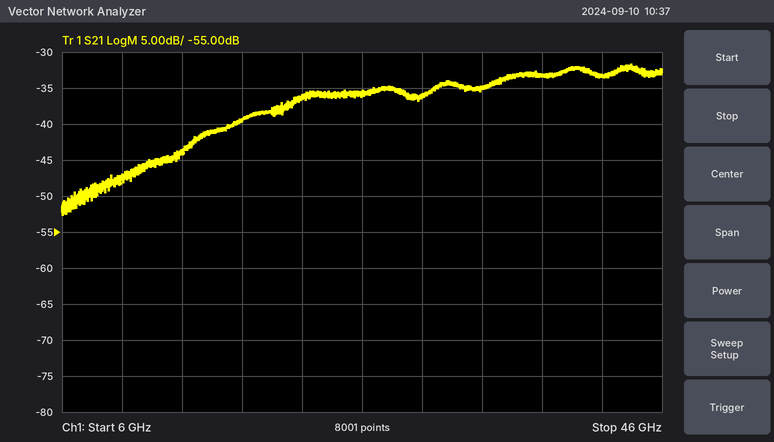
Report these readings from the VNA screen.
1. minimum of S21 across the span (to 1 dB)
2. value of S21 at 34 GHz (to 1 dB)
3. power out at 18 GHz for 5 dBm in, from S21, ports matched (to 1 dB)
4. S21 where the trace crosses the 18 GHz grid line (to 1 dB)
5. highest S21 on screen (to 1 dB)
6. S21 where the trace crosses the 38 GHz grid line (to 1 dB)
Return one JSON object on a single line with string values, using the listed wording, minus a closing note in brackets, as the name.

{"minimum of S21 across the span": "-53 dB", "value of S21 at 34 GHz": "-35 dB", "power out at 18 GHz for 5 dBm in, from S21, ports matched": "-34 dBm", "S21 where the trace crosses the 18 GHz grid line": "-39 dB", "highest S21 on screen": "-32 dB", "S21 where the trace crosses the 38 GHz grid line": "-33 dB"}
